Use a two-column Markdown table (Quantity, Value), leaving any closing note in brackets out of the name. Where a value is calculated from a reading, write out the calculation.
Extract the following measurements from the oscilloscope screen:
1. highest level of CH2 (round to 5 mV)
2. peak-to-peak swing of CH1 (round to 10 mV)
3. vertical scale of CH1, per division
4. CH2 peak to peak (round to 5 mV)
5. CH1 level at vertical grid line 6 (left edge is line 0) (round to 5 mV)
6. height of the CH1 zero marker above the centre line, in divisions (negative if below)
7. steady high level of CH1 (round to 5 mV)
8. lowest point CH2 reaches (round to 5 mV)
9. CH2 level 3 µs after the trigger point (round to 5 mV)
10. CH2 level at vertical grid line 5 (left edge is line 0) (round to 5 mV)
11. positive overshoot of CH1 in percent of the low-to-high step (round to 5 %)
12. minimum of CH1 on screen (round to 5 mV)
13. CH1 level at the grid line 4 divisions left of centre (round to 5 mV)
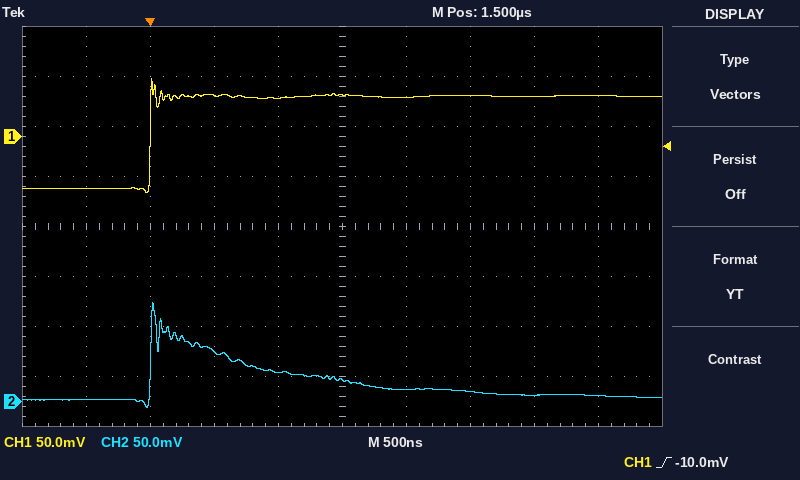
| Quantity | Value |
|---|---|
| highest level of CH2 | 100 mV |
| peak-to-peak swing of CH1 | 110 mV |
| vertical scale of CH1, per division | 50 mV |
| CH2 peak to peak | 100 mV − (-5 mV) = 105 mV |
| CH1 level at vertical grid line 6 (left edge is line 0) | 40 mV |
| height of the CH1 zero marker above the centre line, in divisions | +1.8 div |
| steady high level of CH1 | 40 mV |
| lowest point CH2 reaches | -5 mV |
| CH2 level 3 µs after the trigger point | 5 mV |
| CH2 level at vertical grid line 5 (left edge is line 0) | 20 mV |
| positive overshoot of CH1 in percent of the low-to-high step | 20 % |
| minimum of CH1 on screen | -55 mV |
| CH1 level at the grid line 4 divisions left of centre | -50 mV |
